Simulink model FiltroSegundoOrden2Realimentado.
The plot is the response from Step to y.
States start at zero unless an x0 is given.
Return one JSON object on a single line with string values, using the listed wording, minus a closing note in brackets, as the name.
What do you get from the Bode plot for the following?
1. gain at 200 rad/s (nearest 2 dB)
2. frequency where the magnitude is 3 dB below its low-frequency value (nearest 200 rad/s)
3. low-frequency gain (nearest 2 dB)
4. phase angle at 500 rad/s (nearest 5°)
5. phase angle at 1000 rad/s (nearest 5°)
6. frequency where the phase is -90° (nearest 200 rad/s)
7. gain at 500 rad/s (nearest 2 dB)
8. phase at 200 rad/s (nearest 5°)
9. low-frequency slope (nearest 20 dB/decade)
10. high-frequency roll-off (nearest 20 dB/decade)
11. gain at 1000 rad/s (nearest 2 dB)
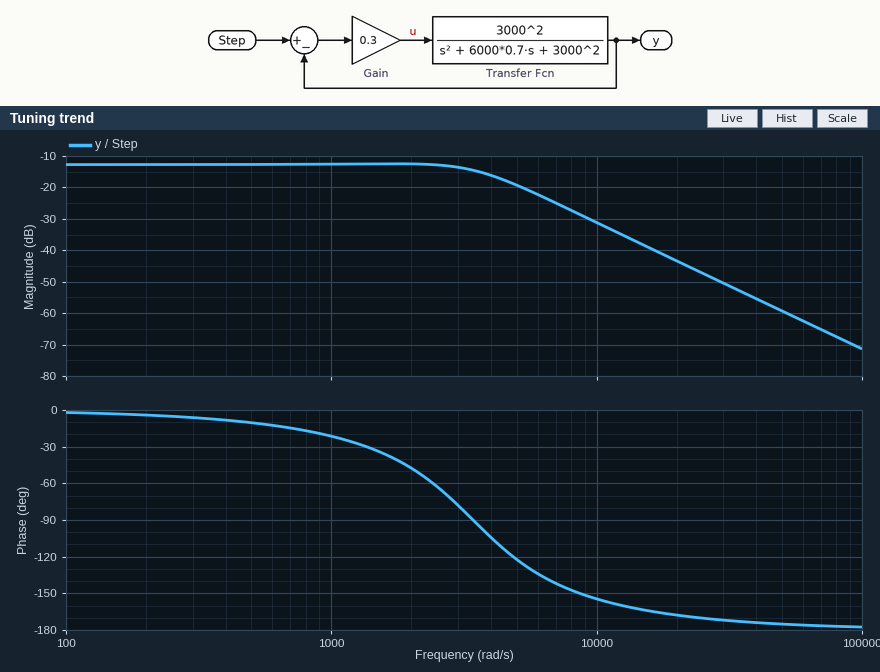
{"gain at 200 rad/s": "-12 dB", "frequency where the magnitude is 3 dB below its low-frequency value": "3800 rad/s", "low-frequency gain": "-12 dB", "phase angle at 500 rad/s": "-10°", "phase angle at 1000 rad/s": "-20°", "frequency where the phase is -90°": "3400 rad/s", "gain at 500 rad/s": "-12 dB", "phase at 200 rad/s": "-5°", "low-frequency slope": "0 dB/decade", "high-frequency roll-off": "-40 dB/decade", "gain at 1000 rad/s": "-12 dB"}
